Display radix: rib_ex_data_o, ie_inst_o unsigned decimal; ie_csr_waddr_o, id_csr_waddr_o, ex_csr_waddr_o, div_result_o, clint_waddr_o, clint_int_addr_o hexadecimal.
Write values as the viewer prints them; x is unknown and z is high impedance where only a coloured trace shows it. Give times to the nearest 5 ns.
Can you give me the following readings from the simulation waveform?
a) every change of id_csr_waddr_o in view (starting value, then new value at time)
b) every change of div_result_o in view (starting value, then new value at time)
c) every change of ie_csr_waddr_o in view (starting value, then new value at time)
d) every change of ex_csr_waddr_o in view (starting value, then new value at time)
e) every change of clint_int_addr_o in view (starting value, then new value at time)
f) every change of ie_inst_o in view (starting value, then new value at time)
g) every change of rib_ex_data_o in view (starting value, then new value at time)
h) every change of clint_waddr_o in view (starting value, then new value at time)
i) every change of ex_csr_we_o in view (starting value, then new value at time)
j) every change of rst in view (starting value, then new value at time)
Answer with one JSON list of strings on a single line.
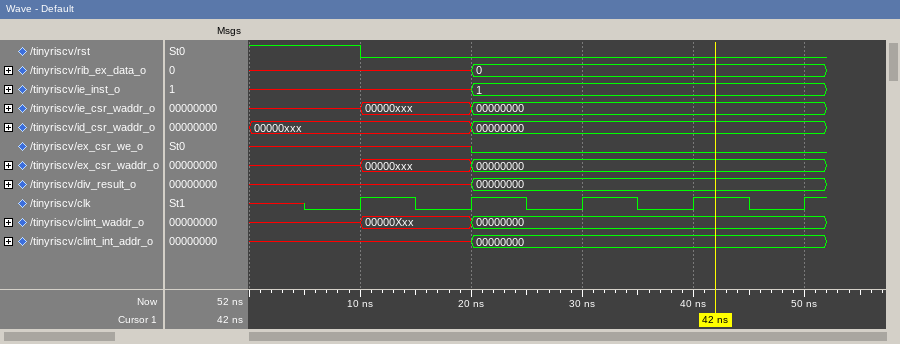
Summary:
["00000xxx, 00000000 at 20 ns", "x, 00000000 at 20 ns", "x, 00000xxx at 10 ns, 00000000 at 20 ns", "x, 00000xxx at 10 ns, 00000000 at 20 ns", "x, 00000000 at 20 ns", "x, 1 at 20 ns", "x, 0 at 20 ns", "x, 00000Xxx at 10 ns, 00000000 at 20 ns", "x, 0 at 20 ns", "1, 0 at 10 ns"]
